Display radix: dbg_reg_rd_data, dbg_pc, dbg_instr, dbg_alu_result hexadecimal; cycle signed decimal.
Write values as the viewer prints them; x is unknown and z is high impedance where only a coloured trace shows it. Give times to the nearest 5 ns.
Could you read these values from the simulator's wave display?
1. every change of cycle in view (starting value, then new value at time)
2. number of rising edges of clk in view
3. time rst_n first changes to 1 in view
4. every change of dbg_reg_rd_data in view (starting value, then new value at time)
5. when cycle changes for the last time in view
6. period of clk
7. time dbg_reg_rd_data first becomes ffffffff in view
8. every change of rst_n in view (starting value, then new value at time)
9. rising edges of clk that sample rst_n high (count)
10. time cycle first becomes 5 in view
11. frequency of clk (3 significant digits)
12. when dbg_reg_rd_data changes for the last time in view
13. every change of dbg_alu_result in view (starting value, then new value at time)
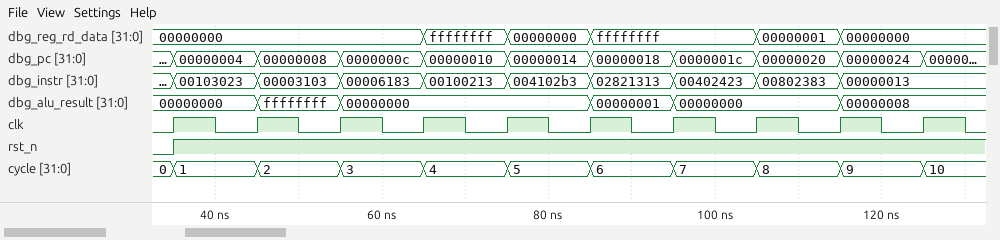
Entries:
0, 1 at 35 ns, 2 at 45 ns, 3 at 55 ns, 4 at 65 ns, 5 at 75 ns, 6 at 85 ns, 7 at 95 ns, 8 at 105 ns, 9 at 115 ns, 10 at 125 ns
10
35 ns
00000000, ffffffff at 65 ns, 00000000 at 75 ns, ffffffff at 85 ns, 00000001 at 105 ns, 00000000 at 115 ns
125 ns
10 ns
65 ns
0, 1 at 35 ns
9
75 ns
100 MHz
115 ns
00000000, ffffffff at 45 ns, 00000000 at 55 ns, 00000001 at 85 ns, 00000000 at 95 ns, 00000008 at 115 ns
